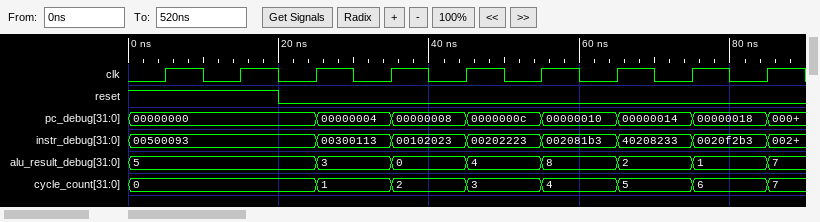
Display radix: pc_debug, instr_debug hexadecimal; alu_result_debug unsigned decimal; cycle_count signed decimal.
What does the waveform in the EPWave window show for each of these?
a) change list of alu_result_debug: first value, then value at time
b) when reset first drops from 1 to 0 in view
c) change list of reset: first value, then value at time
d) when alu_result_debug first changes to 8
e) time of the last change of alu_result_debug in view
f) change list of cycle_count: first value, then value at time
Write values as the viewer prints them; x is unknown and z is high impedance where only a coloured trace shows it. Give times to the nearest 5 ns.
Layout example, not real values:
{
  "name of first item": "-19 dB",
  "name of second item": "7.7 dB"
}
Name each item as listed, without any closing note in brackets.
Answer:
{
  "change list of alu_result_debug: first value, then value at time": "5, 3 at 25 ns, 0 at 35 ns, 4 at 45 ns, 8 at 55 ns, 2 at 65 ns, 1 at 75 ns, 7 at 85 ns",
  "when reset first drops from 1 to 0 in view": "20 ns",
  "change list of reset: first value, then value at time": "1, 0 at 20 ns",
  "when alu_result_debug first changes to 8": "55 ns",
  "time of the last change of alu_result_debug in view": "85 ns",
  "change list of cycle_count: first value, then value at time": "0, 1 at 25 ns, 2 at 35 ns, 3 at 45 ns, 4 at 55 ns, 5 at 65 ns, 6 at 75 ns, 7 at 85 ns"
}
